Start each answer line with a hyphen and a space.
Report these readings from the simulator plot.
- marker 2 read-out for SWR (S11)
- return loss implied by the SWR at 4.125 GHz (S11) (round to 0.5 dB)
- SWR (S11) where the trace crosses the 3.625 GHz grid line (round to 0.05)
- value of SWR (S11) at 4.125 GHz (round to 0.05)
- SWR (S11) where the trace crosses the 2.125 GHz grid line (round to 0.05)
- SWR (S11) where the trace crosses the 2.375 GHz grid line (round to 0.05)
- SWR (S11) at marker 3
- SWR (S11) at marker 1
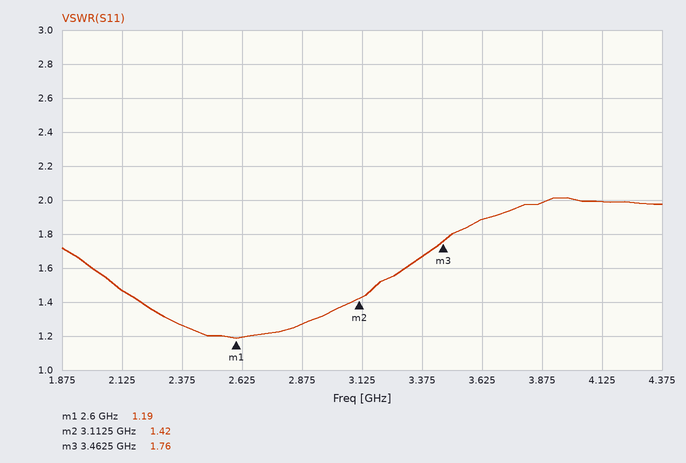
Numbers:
- 1.42
- 9.5 dB
- 1.90
- 2.00
- 1.45
- 1.25
- 1.76
- 1.19
